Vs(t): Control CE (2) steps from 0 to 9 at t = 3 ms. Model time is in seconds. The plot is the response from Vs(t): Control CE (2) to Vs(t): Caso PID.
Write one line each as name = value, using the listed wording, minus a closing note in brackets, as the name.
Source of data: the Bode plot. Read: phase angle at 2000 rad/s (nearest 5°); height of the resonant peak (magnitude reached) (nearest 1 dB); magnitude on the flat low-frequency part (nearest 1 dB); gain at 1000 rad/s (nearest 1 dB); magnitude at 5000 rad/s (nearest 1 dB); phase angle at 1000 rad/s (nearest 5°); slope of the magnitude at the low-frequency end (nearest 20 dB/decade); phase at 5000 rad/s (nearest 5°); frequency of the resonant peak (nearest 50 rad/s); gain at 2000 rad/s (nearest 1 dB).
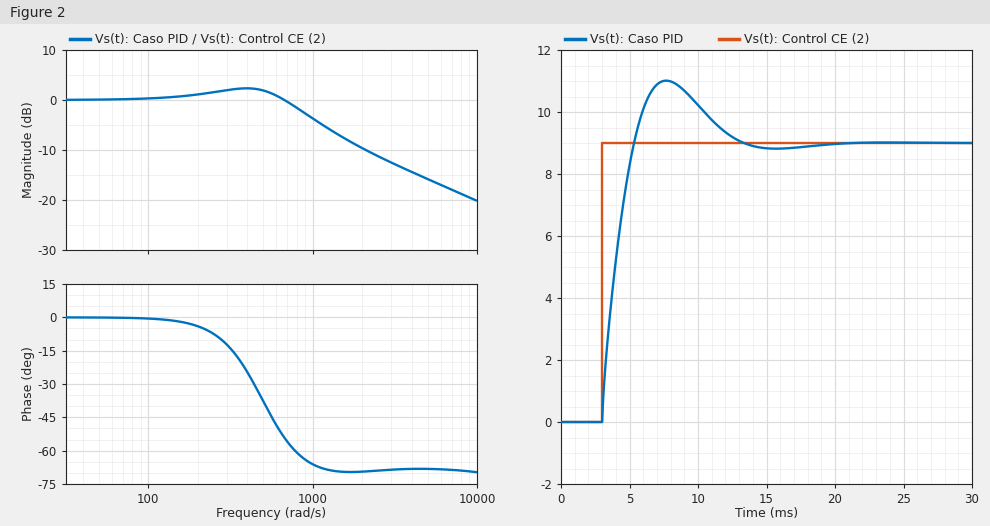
phase angle at 2000 rad/s = -70°
height of the resonant peak (magnitude reached) = 2 dB
magnitude on the flat low-frequency part = 0 dB
gain at 1000 rad/s = -4 dB
magnitude at 5000 rad/s = -16 dB
phase angle at 1000 rad/s = -65°
slope of the magnitude at the low-frequency end = 0 dB/decade
phase at 5000 rad/s = -70°
frequency of the resonant peak = 400 rad/s
gain at 2000 rad/s = -10 dB
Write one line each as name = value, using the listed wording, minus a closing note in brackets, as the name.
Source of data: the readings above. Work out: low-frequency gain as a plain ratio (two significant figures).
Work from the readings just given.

low-frequency gain as a plain ratio = 1.0
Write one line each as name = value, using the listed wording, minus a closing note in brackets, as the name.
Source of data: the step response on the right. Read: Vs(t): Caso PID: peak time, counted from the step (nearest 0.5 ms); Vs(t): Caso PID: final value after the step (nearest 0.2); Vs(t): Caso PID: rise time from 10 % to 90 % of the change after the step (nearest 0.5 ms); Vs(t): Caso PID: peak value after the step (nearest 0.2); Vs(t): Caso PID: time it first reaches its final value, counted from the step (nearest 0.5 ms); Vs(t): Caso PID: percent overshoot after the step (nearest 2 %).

Vs(t): Caso PID: peak time, counted from the step = 4.5 ms
Vs(t): Caso PID: final value after the step = 9.0
Vs(t): Caso PID: rise time from 10 % to 90 % of the change after the step = 2.0 ms
Vs(t): Caso PID: peak value after the step = 11.0
Vs(t): Caso PID: time it first reaches its final value, counted from the step = 2.5 ms
Vs(t): Caso PID: percent overshoot after the step = 22 %
